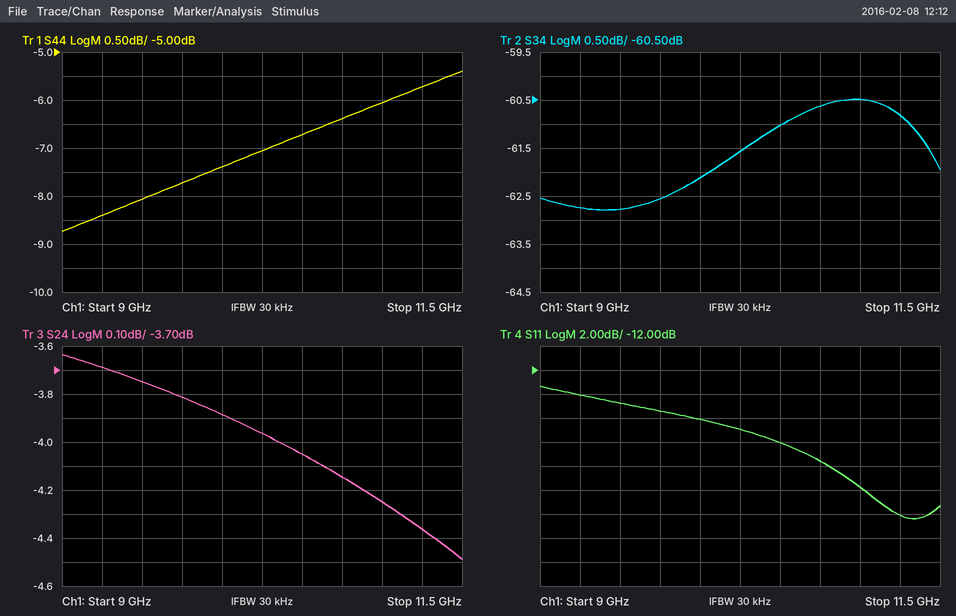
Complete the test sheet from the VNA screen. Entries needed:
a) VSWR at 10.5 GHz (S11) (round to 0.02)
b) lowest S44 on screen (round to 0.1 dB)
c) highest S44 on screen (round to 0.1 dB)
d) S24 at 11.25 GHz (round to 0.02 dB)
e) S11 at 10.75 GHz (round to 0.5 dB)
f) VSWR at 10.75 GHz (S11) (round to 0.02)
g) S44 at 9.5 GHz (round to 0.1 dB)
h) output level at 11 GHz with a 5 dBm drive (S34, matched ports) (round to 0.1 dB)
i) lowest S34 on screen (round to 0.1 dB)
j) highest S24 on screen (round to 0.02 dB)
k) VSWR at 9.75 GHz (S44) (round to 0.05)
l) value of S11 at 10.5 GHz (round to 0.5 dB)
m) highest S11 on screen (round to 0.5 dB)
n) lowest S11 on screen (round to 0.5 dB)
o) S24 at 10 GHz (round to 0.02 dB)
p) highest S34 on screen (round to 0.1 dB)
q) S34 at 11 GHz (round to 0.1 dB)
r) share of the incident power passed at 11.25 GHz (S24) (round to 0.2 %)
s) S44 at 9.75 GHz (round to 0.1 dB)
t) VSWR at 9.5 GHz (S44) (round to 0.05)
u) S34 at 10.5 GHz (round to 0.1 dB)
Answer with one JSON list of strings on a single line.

["1.28", "-8.7 dB", "-5.4 dB", "-4.36 dB", "-19.5 dB", "1.24", "-8.1 dB", "-55.5 dBm", "-62.8 dB", "-3.64 dB", "2.40", "-18.0 dB", "-13.5 dB", "-24.5 dB", "-3.88 dB", "-60.5 dB", "-60.5 dB", "36.6 %", "-7.7 dB", "2.30", "-61.0 dB"]
